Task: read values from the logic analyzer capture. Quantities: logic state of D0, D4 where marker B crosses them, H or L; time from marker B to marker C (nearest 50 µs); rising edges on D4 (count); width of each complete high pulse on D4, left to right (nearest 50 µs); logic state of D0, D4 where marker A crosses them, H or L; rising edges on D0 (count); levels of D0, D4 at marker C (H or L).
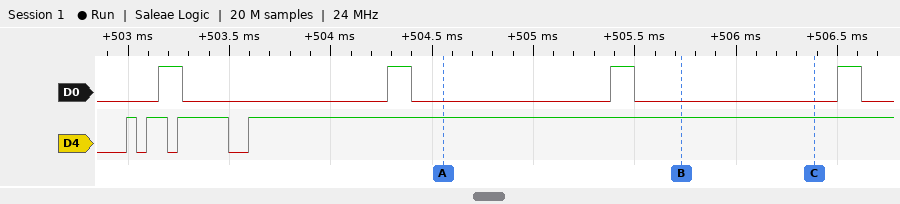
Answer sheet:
D0=L, D4=H
650 µs
4
50 µs, 100 µs, 250 µs
D0=L, D4=H
4
D0=L, D4=H
